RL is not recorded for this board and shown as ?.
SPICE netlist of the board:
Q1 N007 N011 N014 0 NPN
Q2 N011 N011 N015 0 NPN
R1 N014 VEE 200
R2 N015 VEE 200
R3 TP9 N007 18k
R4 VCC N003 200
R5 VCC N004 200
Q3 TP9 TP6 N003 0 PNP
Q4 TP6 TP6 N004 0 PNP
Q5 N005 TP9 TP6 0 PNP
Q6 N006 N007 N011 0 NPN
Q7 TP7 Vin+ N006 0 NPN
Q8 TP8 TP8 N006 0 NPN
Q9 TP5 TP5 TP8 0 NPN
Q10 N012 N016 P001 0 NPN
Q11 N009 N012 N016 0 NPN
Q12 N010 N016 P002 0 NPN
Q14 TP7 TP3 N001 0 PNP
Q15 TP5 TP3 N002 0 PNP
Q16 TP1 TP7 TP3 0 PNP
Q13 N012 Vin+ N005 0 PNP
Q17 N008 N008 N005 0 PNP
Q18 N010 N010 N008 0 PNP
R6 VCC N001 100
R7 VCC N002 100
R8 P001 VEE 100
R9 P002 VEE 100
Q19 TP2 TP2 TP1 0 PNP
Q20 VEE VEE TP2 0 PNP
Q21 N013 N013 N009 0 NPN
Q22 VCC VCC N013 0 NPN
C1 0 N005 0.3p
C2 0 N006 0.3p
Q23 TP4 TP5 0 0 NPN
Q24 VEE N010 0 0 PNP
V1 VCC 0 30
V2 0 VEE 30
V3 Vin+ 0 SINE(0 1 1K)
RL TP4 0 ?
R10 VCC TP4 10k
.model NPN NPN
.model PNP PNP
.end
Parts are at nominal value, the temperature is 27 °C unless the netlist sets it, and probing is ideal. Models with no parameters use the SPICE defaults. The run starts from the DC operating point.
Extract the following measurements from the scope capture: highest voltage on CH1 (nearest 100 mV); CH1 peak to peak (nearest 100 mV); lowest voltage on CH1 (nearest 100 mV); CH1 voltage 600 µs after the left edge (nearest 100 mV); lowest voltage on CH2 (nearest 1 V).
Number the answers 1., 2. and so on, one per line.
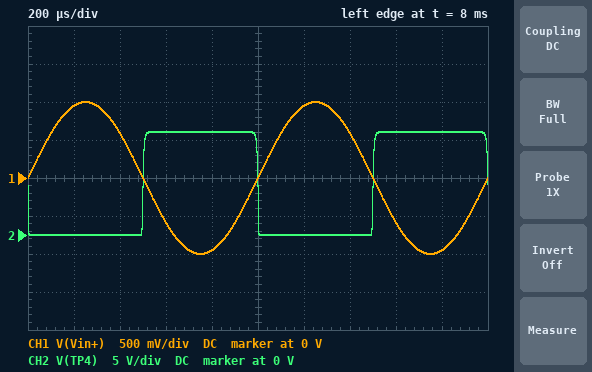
1. 1.0 V
2. 2.0 V
3. -1.0 V
4. -600 mV
5. 0 V
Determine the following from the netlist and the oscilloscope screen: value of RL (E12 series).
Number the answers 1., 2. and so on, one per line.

1. 8.2 kΩ
